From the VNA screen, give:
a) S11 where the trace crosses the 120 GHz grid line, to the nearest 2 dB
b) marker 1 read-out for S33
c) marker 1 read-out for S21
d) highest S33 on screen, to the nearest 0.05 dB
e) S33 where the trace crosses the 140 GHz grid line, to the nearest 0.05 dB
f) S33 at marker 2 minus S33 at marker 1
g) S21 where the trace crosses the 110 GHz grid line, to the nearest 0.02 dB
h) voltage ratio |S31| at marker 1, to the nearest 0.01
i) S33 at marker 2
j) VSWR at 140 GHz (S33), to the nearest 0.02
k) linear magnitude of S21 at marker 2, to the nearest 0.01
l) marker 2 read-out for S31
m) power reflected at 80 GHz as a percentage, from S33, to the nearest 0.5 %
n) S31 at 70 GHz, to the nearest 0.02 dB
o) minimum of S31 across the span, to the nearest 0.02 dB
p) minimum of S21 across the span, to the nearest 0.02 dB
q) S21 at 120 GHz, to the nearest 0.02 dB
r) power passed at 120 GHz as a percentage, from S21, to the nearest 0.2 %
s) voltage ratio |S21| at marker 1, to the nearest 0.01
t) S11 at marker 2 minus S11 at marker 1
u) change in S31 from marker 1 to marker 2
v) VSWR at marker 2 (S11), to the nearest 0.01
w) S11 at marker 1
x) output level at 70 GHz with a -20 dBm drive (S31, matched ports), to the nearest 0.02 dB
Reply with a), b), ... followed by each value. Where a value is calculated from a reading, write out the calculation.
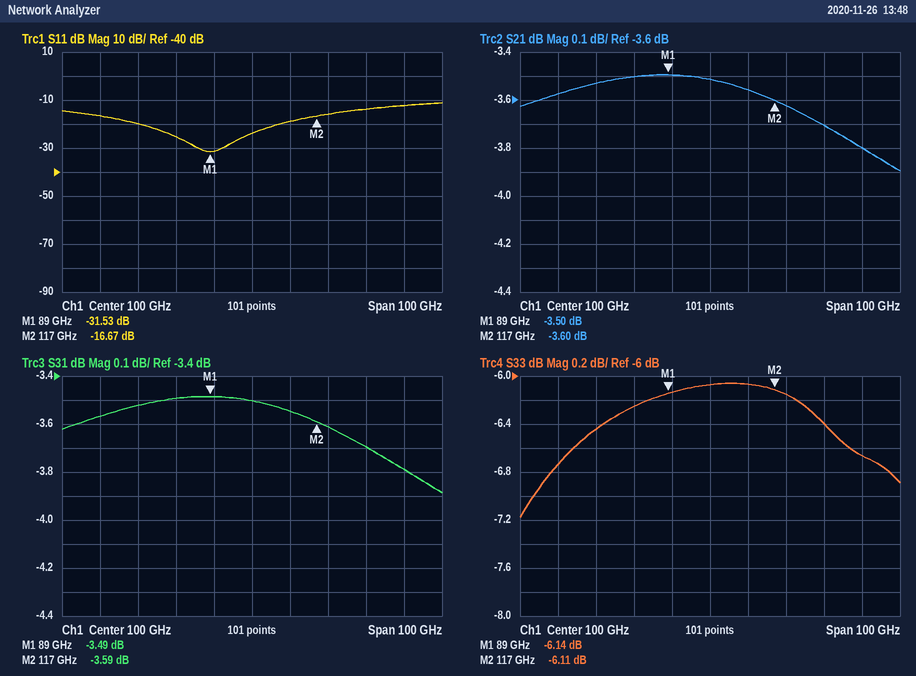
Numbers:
a) -16 dB
b) -6.14 dB
c) -3.50 dB
d) -6.05 dB
e) -6.65 dB
f) -6.11 − (-6.14) = 0.03 dB
g) -3.56 dB
h) 10^(-3.49/20) ≈ 0.67
i) -6.11 dB
j) |Γ| = 10^(-6.65/20) = 0.4651; VSWR = (1 + 0.4651)/(1 − 0.4651) ≈ 2.74
k) 10^(-3.6/20) ≈ 0.66
l) -3.59 dB
m) 10^(-6.25/10) ≈ 23.7 %, so 23.5 % to the nearest 0.5 %
n) -3.52 dB
o) -3.88 dB
p) -3.90 dB
q) -3.62 dB
r) 10^(-3.62/10) ≈ 43.5 %, so 43.4 % to the nearest 0.2 %
s) 10^(-3.5/20) ≈ 0.67
t) -16.67 − (-31.53) = 14.86 dB
u) -3.59 − (-3.49) = -0.10 dB
v) (1 + 0.1467)/(1 − 0.1467) ≈ 1.34
w) -31.53 dB
x) -20 dBm + (-3.52 dB) = -23.52 dBm
